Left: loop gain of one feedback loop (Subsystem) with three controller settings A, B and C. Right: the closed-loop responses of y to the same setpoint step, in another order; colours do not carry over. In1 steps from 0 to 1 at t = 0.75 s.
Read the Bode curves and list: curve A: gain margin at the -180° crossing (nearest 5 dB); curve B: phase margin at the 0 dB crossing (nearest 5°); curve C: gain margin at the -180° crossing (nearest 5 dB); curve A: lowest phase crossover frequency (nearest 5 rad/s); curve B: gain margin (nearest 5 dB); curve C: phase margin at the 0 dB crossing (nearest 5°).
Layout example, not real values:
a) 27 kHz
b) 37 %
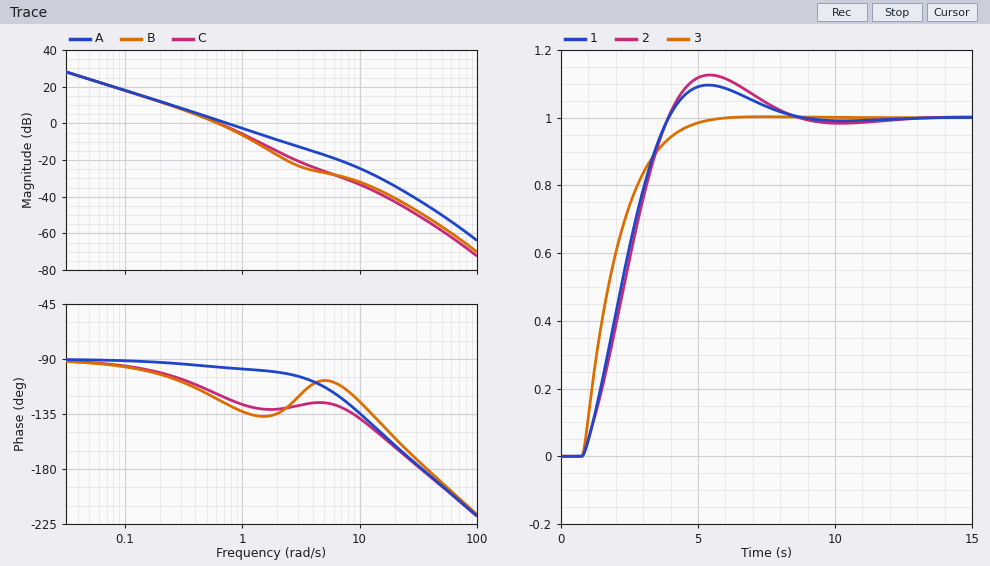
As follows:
a) 45 dB
b) 55°
c) 50 dB
d) 35 rad/s
e) 50 dB
f) 60°
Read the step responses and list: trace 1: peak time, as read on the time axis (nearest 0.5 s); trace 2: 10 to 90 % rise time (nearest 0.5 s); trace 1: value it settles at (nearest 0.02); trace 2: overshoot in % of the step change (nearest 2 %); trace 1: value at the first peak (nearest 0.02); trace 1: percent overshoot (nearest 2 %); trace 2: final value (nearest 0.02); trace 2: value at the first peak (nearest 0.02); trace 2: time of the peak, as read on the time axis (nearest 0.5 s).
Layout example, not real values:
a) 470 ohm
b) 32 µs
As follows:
a) 5.5 s
b) 2.5 s
c) 1.00
d) 12 %
e) 1.10
f) 10 %
g) 1.00
h) 1.12
i) 5.5 s
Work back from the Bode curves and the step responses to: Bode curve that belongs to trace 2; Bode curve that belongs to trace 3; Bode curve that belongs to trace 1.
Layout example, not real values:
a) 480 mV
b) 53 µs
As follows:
a) B
b) A
c) C
